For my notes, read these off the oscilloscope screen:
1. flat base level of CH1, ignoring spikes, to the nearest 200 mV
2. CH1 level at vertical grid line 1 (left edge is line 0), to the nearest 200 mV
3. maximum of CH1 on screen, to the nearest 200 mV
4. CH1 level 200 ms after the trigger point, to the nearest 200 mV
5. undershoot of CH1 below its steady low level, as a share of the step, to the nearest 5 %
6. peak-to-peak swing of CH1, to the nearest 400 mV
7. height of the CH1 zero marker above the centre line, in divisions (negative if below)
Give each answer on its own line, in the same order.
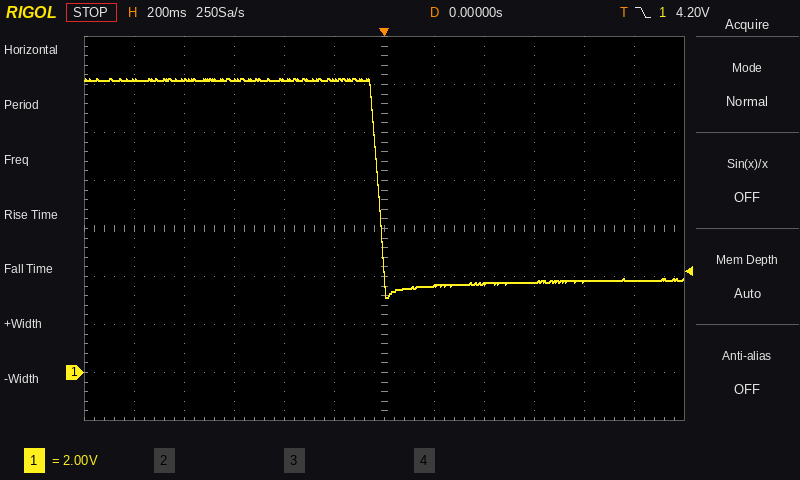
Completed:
3.8 V
12.2 V
12.2 V
3.6 V
10 %
9.2 V
-3.0 div
